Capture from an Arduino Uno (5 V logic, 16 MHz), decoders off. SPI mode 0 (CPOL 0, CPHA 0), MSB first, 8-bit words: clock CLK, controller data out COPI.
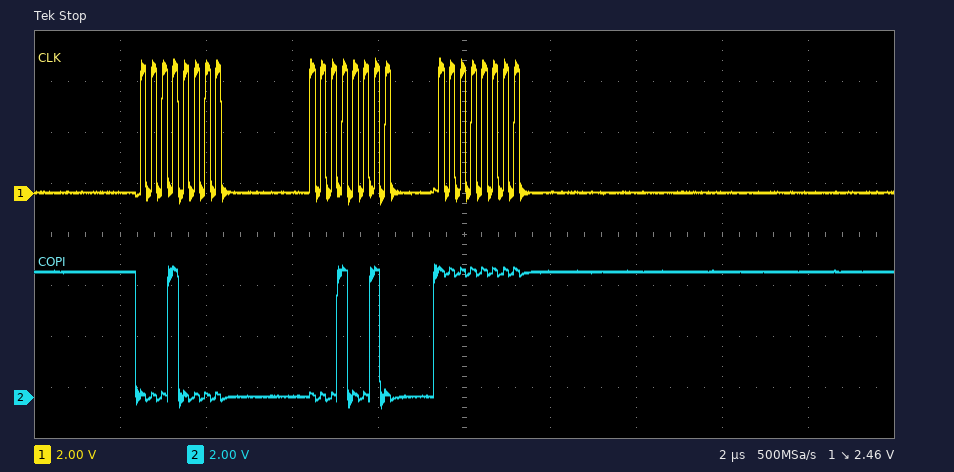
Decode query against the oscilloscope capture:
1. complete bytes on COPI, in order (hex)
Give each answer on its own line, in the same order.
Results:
10 12 FF
